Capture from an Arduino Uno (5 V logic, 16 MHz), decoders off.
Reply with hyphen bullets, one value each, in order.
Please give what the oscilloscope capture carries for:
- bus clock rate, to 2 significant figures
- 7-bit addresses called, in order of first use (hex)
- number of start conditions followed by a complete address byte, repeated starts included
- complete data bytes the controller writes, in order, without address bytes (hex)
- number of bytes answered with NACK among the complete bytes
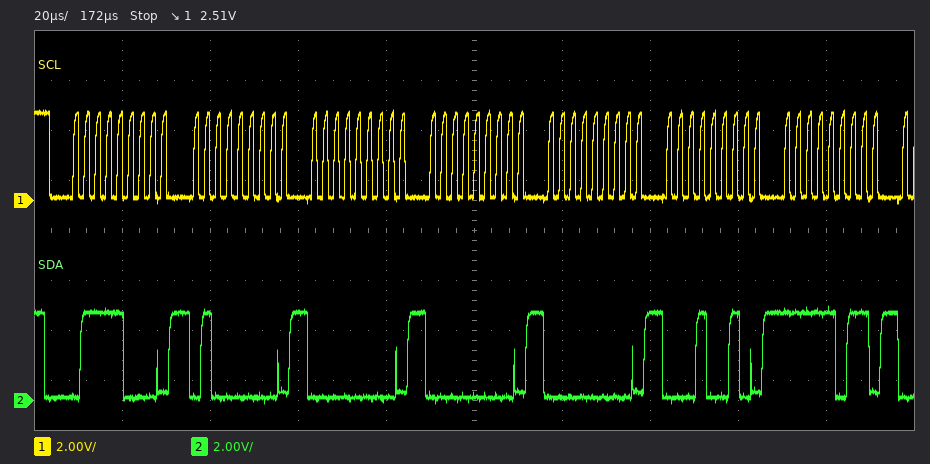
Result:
- 400 kHz
- 0x3C
- 1
- 40 00 00 00 12 FB
- 0
